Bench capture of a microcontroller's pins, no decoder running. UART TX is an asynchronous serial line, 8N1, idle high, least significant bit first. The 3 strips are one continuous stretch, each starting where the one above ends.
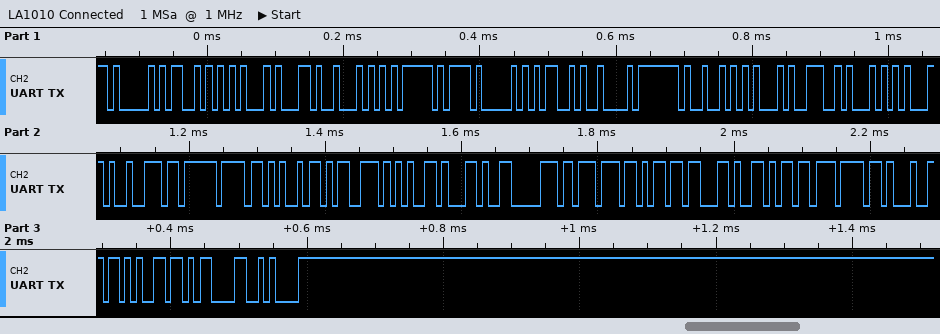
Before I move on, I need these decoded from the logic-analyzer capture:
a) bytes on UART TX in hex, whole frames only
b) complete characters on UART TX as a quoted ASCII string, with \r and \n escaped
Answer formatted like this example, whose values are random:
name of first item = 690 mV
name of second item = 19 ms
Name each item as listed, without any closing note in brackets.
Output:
bytes on UART TX in hex, whole frames only = 41 53 45 2C 54 5F 41 4D 42 49 45 4E 54 2C 6E 6F 69 73 65 2C 70 77 6D 2C 6D 6F 64 65 0D 0A
complete characters on UART TX as a quoted ASCII string, with \r and \n escaped = "ASE,T_AMBIENT,noise,pwm,mode\r\n"
